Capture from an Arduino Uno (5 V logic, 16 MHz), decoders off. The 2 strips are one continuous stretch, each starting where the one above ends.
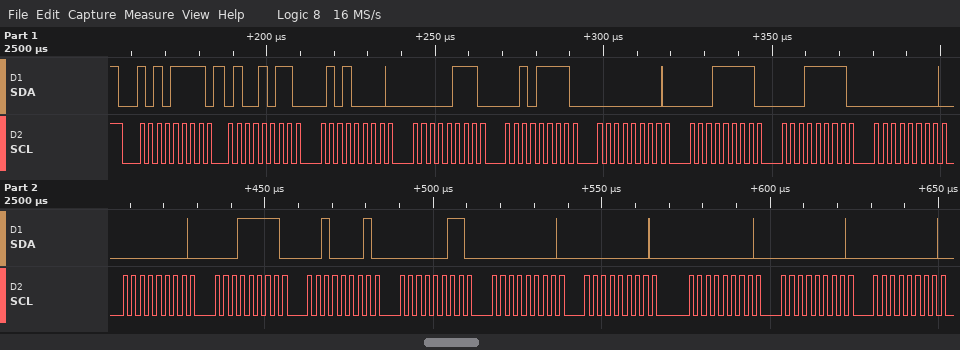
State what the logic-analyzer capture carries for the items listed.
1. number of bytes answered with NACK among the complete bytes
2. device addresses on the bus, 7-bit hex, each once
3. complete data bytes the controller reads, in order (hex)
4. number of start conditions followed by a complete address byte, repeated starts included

0
0x57
4B 50 07 2F 00 1F 1F 00 00 1F 21 03 00 00 00 00 00
1
